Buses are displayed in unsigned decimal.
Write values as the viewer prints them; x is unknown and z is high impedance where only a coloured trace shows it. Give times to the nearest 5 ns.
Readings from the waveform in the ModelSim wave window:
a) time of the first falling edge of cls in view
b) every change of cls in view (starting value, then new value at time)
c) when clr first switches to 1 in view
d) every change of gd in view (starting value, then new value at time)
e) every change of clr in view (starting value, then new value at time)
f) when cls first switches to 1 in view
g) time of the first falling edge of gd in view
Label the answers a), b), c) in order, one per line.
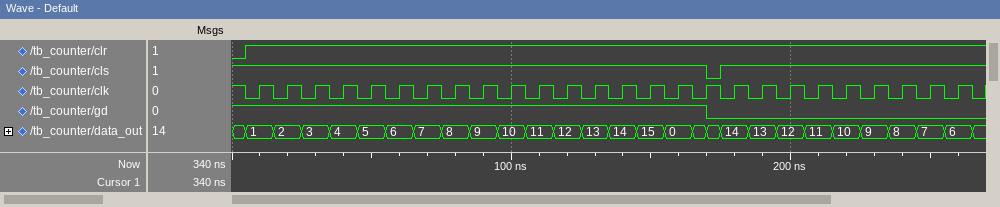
a) 170 ns
b) 1, 0 at 170 ns, 1 at 175 ns
c) 5 ns
d) 1, 0 at 170 ns
e) 0, 1 at 5 ns
f) 175 ns
g) 170 ns
